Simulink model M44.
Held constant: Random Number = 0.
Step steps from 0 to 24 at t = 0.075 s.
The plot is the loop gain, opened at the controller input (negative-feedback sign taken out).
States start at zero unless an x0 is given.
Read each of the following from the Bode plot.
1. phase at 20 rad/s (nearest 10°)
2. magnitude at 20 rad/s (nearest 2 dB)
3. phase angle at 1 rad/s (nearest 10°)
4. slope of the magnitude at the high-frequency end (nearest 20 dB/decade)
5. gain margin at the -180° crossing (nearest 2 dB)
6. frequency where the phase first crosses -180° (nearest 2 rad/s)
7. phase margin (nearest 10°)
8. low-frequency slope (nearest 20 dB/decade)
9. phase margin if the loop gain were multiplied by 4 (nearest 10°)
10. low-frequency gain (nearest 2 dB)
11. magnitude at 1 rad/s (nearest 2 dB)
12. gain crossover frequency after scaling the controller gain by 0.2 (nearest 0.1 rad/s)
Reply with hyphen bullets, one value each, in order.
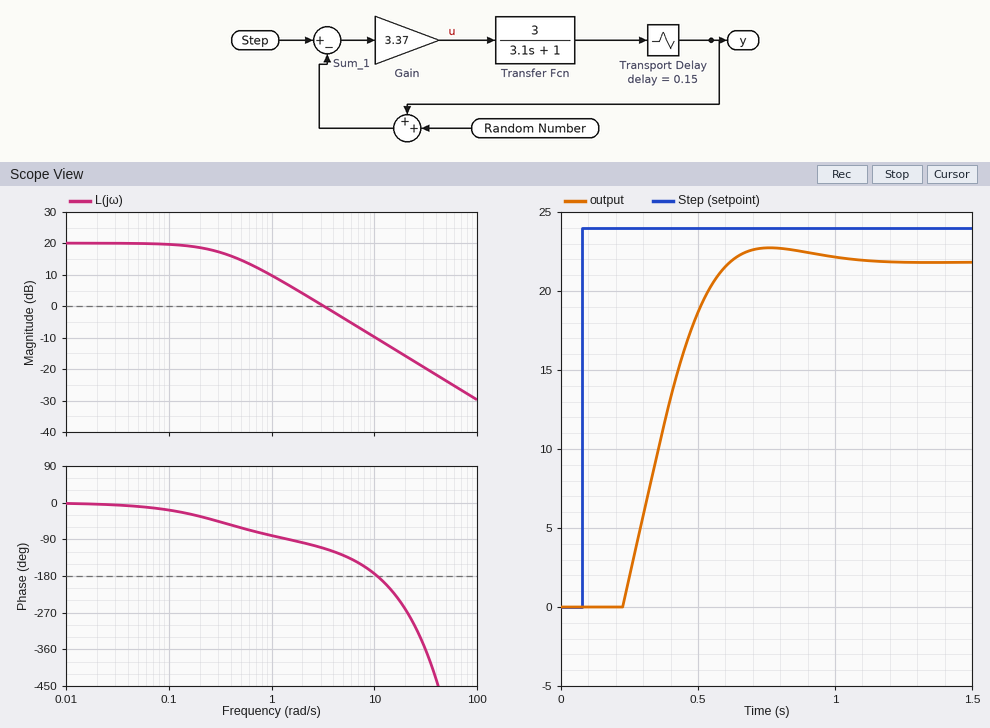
- -260°
- -16 dB
- -80°
- -20 dB/decade
- 10 dB
- 10 rad/s
- 70°
- 0 dB/decade
- -20°
- 20 dB
- 10 dB
- 0.6 rad/s
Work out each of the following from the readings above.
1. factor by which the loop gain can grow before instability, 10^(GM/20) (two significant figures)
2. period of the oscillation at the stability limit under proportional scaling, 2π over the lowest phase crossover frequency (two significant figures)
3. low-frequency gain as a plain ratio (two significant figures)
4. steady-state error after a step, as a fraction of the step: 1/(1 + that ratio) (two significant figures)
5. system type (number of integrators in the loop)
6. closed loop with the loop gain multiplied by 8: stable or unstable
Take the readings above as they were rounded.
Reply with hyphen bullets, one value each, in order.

- 3.2
- 0.63 s
- 10
- 0.091
- 0
- unstable
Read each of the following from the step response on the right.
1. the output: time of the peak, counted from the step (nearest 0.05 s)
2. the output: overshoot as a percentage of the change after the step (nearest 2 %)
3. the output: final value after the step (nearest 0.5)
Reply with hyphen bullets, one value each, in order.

- 0.70 s
- 4 %
- 22.0
